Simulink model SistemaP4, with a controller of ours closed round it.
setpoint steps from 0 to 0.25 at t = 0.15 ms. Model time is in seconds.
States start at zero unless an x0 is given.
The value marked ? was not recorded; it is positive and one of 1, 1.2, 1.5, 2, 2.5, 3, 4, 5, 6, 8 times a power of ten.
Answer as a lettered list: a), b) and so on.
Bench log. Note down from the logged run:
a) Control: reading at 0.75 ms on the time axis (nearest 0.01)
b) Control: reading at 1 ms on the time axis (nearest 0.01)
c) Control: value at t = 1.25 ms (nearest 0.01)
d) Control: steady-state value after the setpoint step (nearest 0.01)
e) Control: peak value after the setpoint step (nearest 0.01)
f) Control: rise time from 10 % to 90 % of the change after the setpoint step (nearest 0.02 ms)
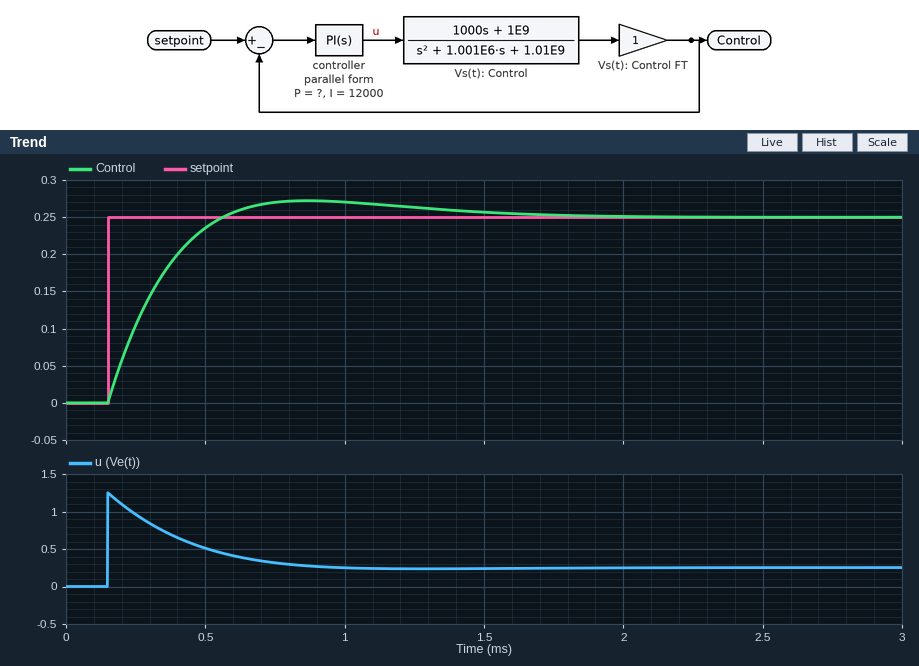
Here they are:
a) 0.27
b) 0.27
c) 0.26
d) 0.25
e) 0.27
f) 0.30 ms
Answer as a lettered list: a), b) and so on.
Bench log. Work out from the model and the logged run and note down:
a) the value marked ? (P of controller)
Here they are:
a) 5
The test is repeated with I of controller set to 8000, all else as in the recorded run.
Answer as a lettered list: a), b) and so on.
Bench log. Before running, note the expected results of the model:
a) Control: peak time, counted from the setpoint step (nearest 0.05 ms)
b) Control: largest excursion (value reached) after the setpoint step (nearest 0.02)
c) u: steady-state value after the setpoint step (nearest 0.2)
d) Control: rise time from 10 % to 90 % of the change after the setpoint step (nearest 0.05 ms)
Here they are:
a) 0.90 ms
b) 0.26
c) 0.2
d) 0.35 ms
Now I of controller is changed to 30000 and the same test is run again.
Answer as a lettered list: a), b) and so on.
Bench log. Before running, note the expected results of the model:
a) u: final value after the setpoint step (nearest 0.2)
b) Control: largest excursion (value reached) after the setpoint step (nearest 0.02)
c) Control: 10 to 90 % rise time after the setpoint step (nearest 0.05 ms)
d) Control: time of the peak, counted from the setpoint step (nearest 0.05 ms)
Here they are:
a) 0.2
b) 0.30
c) 0.20 ms
d) 0.45 ms
